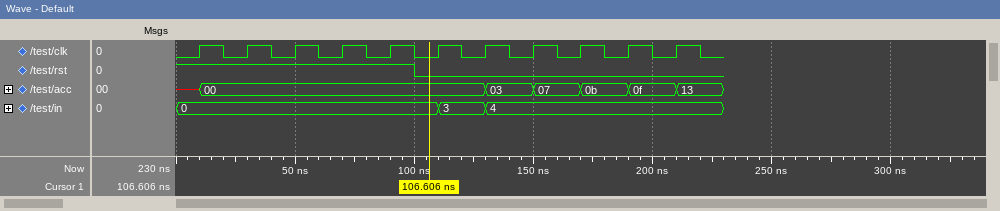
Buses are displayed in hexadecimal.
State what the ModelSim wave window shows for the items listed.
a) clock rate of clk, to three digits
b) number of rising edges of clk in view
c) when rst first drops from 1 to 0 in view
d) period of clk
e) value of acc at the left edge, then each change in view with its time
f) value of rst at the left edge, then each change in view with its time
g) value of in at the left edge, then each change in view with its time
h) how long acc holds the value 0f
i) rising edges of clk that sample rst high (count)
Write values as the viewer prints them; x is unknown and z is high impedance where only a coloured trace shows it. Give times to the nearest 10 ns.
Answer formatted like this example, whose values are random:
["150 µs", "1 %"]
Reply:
["50.0 MHz", "11", "100 ns", "20 ns", "x, 00 at 10 ns, 03 at 130 ns, 07 at 150 ns, 0b at 170 ns, 0f at 190 ns, 13 at 210 ns", "1, 0 at 100 ns", "0, 3 at 110 ns, 4 at 130 ns", "20 ns", "5"]
